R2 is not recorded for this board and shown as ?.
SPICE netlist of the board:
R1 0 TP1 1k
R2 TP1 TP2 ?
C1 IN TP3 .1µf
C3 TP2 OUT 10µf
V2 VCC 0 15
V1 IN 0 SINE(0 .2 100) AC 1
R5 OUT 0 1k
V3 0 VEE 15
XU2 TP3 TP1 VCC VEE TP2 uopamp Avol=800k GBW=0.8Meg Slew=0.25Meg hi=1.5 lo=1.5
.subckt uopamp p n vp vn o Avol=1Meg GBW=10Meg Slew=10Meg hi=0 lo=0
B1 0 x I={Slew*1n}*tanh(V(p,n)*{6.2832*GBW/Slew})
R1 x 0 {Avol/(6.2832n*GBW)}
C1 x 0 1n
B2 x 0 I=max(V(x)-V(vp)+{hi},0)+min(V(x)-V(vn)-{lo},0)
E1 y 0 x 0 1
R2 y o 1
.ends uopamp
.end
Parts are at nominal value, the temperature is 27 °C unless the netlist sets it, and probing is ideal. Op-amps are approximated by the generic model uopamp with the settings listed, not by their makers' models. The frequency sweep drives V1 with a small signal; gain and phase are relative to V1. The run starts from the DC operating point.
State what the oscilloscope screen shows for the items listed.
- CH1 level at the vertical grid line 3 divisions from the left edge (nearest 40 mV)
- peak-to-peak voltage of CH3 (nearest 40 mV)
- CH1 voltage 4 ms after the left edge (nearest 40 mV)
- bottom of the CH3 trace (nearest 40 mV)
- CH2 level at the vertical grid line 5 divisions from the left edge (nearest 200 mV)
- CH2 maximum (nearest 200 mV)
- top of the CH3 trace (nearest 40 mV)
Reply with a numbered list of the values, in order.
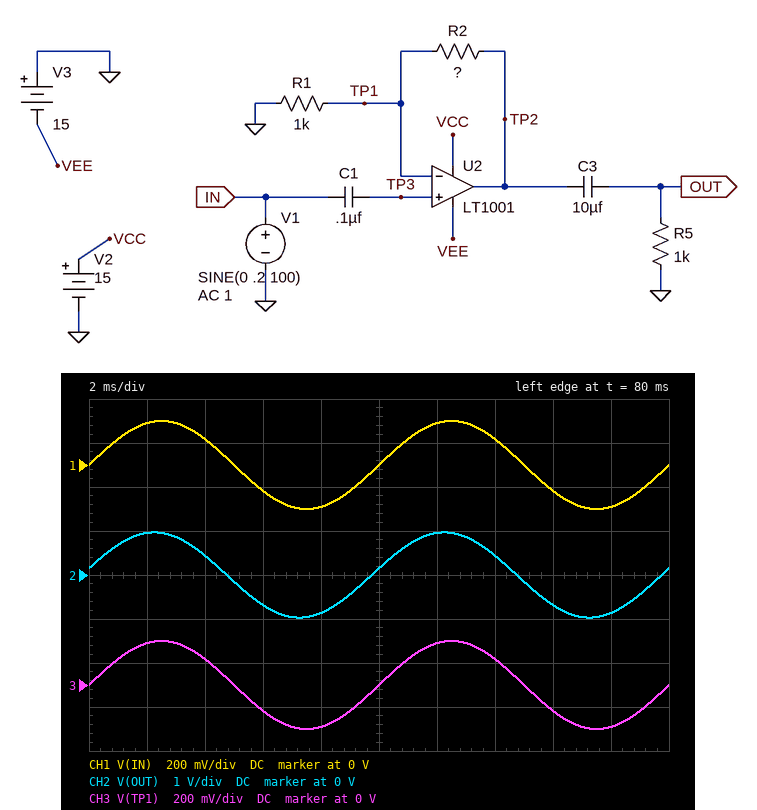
1. -120 mV
2. 400 mV
3. 120 mV
4. -200 mV
5. 200 mV
6. 1.0 V
7. 200 mV
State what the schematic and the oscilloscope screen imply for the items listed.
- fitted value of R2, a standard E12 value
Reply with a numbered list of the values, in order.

1. 3.9 kΩ
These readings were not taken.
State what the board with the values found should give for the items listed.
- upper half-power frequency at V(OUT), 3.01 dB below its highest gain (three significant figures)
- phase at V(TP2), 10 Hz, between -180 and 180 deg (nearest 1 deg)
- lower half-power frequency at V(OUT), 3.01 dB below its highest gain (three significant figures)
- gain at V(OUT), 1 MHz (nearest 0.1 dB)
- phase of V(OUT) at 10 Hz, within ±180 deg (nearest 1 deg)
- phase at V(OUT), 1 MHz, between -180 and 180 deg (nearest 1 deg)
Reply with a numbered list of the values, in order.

1. 163 kHz
2. 0 deg
3. 15.9 Hz
4. -2.1 dB
5. 58 deg
6. -81 deg
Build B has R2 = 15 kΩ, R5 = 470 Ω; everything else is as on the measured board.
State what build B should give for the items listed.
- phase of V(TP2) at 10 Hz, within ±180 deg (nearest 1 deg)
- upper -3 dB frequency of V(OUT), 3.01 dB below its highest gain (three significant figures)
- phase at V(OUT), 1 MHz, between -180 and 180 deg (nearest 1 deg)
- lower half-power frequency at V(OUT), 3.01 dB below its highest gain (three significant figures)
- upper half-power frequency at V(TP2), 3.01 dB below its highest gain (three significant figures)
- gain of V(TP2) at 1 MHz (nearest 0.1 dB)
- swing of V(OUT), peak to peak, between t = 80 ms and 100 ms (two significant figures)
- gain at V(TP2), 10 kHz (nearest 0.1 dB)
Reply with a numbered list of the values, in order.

1. 0 deg
2. 50.0 kHz
3. -87 deg
4. 33.8 Hz
5. 49.9 kHz
6. -2.0 dB
7. 6.1 V
8. 23.9 dB
